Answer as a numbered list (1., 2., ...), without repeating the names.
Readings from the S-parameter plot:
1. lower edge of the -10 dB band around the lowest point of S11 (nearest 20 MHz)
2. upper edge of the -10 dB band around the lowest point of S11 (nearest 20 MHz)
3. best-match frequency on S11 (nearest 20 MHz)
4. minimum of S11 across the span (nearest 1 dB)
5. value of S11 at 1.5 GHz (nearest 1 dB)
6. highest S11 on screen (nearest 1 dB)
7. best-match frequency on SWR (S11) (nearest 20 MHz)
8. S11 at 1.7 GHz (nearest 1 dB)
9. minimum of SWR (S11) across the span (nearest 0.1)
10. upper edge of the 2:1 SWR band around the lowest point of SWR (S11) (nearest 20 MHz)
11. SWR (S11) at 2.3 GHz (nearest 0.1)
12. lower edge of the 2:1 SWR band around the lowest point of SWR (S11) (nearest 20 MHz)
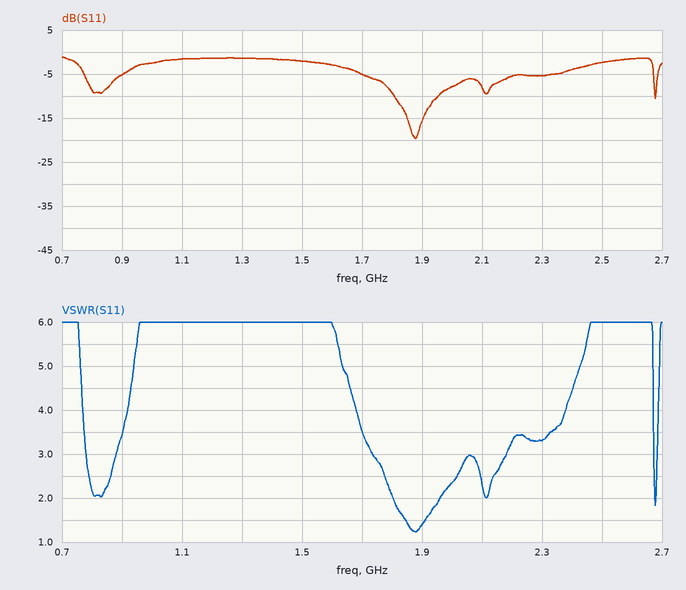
1. 1.80 GHz
2. 1.96 GHz
3. 1.88 GHz
4. -20 dB
5. -2 dB
6. -1 dB
7. 1.88 GHz
8. -5 dB
9. 1.2
10. 1.96 GHz
11. 3.3
12. 1.80 GHz
